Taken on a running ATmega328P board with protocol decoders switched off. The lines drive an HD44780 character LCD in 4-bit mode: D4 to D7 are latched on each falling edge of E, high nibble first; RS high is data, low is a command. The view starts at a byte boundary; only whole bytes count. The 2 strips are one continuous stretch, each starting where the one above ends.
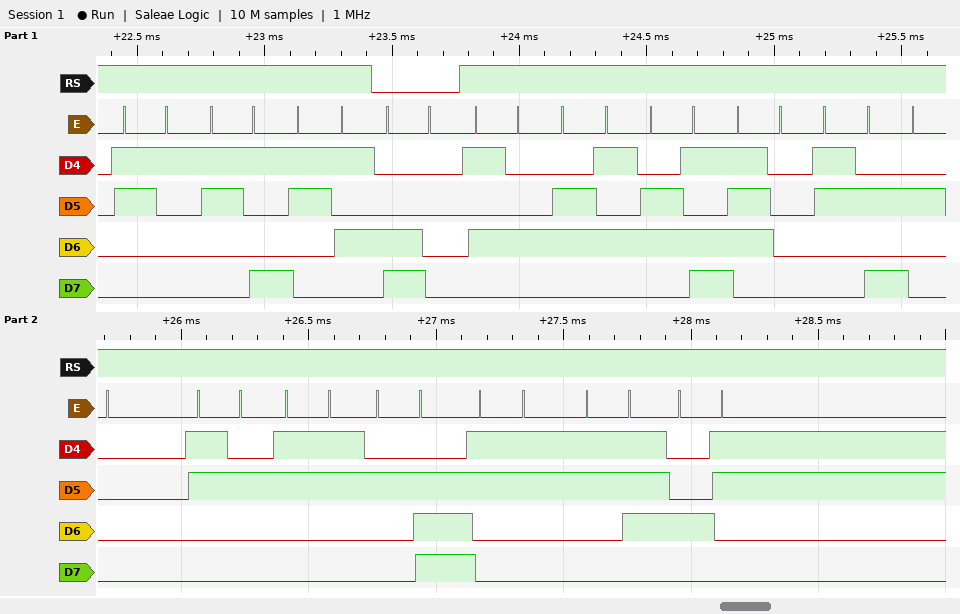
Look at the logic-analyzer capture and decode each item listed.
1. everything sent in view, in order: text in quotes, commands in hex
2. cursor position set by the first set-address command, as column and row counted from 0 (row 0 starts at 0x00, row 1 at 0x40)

"195" 0xC0 "Temp: 23.37C"
column 0, row 1
